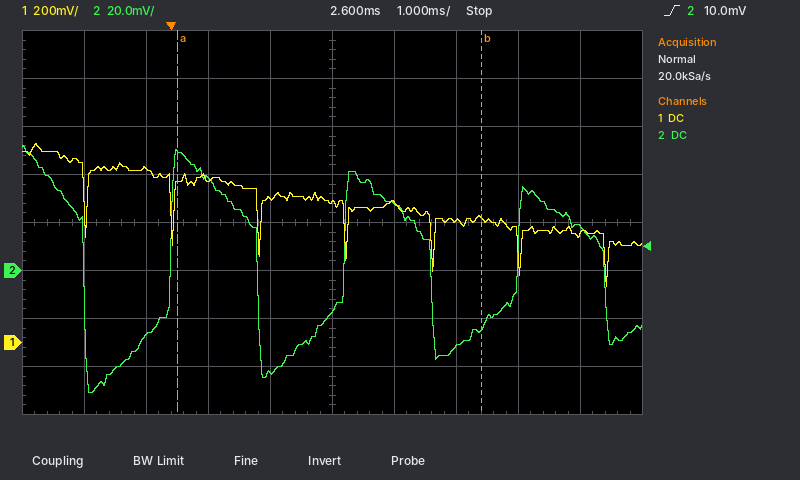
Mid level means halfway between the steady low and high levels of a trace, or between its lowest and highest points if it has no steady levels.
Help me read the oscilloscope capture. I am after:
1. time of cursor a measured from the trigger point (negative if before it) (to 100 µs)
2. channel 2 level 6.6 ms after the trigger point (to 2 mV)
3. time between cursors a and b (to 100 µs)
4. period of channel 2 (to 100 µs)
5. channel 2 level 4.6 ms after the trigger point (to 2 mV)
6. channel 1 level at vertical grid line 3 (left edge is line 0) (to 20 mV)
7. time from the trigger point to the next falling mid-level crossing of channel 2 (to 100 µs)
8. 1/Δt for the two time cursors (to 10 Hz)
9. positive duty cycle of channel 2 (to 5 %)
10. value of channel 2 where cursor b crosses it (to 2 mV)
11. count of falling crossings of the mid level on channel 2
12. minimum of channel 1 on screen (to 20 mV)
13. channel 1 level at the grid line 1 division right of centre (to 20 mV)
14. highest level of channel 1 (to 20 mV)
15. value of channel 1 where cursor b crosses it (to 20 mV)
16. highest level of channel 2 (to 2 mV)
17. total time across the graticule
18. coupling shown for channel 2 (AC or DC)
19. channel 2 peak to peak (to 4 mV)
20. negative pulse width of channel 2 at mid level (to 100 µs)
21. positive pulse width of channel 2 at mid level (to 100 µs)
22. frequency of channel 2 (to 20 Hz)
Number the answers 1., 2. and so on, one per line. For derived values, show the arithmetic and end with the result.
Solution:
1. +100 µs
2. 18 mV
3. 4.9 ms
4. 2.8 ms
5. -32 mV
6. 680 mV
7. 1.4 ms
8. 1 / 4.9 ms ≈ 200 Hz
9. 1.4 ms / 2.8 ms ≈ 50 %
10. -24 mV
11. 4
12. 240 mV
13. 580 mV
14. 820 mV
15. 520 mV
16. 52 mV
17. 10 ms
18. DC
19. 104 mV
20. 1.4 ms
21. 1.4 ms
22. 1 / 2.8 ms ≈ 357 Hz, so 360 Hz to the nearest 20 Hz
